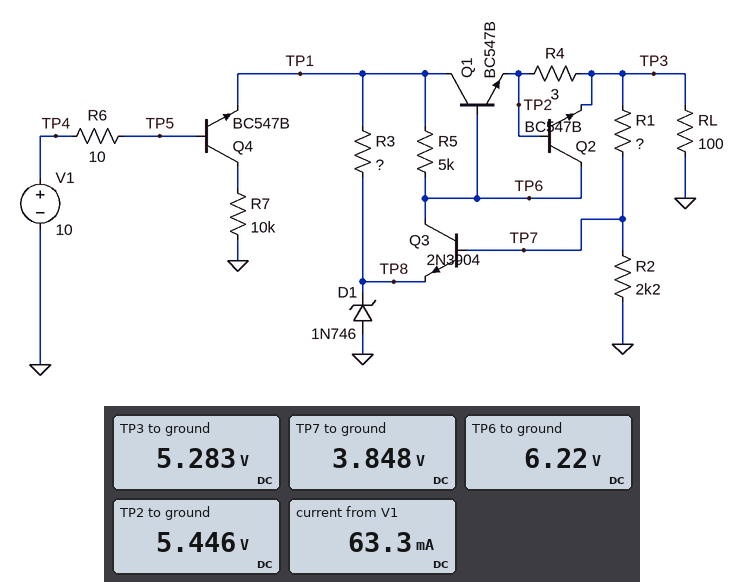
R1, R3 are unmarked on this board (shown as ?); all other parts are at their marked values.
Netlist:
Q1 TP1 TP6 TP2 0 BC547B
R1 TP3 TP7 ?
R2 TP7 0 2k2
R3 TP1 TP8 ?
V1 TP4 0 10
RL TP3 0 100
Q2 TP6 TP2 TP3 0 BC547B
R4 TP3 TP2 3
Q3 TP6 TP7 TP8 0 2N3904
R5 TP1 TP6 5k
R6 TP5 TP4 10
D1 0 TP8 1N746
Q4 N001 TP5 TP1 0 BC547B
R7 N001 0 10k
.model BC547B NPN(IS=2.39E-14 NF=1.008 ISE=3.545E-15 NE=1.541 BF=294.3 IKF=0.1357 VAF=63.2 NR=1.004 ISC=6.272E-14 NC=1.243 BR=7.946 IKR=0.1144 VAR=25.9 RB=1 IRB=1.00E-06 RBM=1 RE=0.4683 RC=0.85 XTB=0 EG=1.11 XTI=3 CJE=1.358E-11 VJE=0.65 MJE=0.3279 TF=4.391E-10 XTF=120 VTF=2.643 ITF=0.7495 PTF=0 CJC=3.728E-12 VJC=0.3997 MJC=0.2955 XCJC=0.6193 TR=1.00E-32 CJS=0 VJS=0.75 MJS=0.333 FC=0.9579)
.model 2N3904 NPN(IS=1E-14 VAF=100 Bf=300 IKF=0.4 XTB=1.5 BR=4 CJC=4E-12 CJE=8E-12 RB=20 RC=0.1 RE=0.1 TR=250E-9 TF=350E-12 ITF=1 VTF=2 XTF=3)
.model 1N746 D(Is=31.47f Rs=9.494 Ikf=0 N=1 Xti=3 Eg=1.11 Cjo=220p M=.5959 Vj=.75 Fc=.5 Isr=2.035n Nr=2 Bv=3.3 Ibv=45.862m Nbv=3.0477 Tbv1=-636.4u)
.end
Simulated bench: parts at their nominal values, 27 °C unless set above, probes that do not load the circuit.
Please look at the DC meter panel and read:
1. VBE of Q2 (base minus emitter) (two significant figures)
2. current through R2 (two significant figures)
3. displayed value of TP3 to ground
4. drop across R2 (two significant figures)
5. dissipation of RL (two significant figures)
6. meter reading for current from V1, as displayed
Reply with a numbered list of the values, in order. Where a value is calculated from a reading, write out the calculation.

1. 5.446 V - 5.283 V = 160 mV
2. (3.848 V) / 2.2 kΩ = 1.7 mA
3. 5.283 V
4. 3.848 V = 3.8 V
5. (5.283 V)^2 / 100 Ω = 280 mW
6. 63.3 mA
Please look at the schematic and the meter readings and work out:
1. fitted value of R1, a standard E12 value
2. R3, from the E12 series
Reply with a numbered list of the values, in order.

1. 820 Ω
2. 680 Ω
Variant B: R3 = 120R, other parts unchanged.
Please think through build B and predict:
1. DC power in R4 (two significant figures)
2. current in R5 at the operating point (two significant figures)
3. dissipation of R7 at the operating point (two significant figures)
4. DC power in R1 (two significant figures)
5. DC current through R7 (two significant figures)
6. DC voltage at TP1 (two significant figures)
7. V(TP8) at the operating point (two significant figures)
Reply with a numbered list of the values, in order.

1. 10 mW
2. 290 µA
3. 6.6 mW
4. 2.9 mW
5. 810 µA
6. 8.1 V
7. 3.6 V
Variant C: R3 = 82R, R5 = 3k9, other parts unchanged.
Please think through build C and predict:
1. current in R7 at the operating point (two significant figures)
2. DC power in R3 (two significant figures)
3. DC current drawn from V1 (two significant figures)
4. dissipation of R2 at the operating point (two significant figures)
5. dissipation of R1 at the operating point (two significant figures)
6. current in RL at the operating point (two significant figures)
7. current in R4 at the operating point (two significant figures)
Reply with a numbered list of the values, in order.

1. 800 µA
2. 210 mW
3. 110 mA
4. 8.1 mW
5. 3.0 mW
6. 58 mA
7. 60 mA
